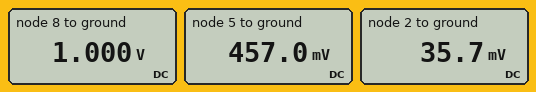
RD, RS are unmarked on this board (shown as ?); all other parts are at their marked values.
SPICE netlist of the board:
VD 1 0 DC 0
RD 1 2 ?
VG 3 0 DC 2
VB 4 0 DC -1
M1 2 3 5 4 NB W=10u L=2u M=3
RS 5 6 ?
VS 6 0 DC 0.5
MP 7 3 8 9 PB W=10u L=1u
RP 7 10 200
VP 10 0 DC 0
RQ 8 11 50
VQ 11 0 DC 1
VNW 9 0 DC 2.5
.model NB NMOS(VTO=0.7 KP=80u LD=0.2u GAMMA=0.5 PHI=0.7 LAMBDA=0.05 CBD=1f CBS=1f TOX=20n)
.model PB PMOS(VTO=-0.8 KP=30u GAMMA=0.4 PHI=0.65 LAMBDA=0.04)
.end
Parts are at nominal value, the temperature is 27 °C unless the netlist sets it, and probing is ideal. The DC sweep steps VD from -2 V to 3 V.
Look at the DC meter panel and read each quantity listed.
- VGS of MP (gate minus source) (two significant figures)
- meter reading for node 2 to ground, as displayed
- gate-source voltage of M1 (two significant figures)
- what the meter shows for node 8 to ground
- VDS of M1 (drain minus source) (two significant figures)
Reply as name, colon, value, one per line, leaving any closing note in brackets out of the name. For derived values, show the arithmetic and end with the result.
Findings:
VGS of MP (gate minus source): 2 V - 1 V = 1.0 V
meter reading for node 2 to ground, as displayed: 35.7 mV
gate-source voltage of M1: 2 V - 457 mV = 1.5 V
what the meter shows for node 8 to ground: 1.000 V
VDS of M1 (drain minus source): 35.7 mV - 457 mV = -420 mV
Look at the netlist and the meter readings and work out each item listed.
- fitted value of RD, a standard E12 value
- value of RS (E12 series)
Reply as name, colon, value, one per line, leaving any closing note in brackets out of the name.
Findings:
fitted value of RD, a standard E12 value: 68 Ω
value of RS: 82 Ω
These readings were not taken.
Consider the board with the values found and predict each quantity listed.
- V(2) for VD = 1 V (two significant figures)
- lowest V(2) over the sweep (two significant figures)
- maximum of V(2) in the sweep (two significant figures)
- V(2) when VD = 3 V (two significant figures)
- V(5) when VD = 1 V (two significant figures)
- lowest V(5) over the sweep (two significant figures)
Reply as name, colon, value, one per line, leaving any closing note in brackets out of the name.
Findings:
V(2) for VD = 1 V: 990 mV
lowest V(2) over the sweep: -1.6 V
maximum of V(2) in the sweep: 3.0 V
V(2) when VD = 3 V: 3.0 V
V(5) when VD = 1 V: 510 mV
lowest V(5) over the sweep: 18 mV
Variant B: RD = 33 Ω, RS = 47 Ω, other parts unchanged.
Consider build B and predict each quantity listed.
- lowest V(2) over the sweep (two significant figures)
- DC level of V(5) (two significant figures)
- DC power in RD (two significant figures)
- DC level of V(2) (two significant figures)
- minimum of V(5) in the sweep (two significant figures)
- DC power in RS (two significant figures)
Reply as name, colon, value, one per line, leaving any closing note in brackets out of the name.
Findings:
lowest V(2) over the sweep: -1.7 V
DC level of V(5): 470 mV
DC power in RD: 11 µW
DC level of V(2): 19 mV
minimum of V(5) in the sweep: 180 mV
DC power in RS: 15 µW
